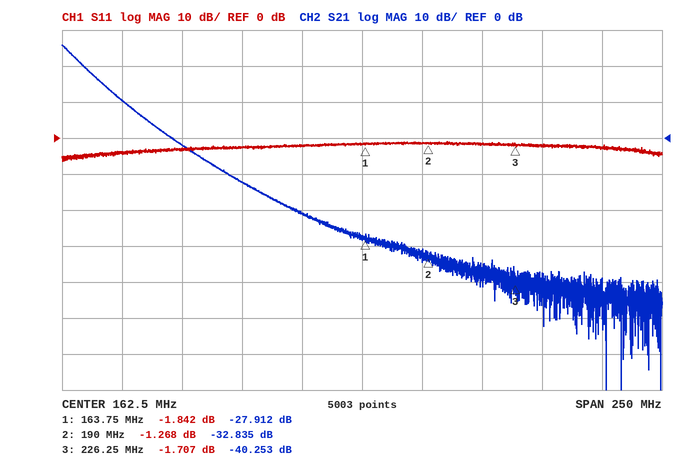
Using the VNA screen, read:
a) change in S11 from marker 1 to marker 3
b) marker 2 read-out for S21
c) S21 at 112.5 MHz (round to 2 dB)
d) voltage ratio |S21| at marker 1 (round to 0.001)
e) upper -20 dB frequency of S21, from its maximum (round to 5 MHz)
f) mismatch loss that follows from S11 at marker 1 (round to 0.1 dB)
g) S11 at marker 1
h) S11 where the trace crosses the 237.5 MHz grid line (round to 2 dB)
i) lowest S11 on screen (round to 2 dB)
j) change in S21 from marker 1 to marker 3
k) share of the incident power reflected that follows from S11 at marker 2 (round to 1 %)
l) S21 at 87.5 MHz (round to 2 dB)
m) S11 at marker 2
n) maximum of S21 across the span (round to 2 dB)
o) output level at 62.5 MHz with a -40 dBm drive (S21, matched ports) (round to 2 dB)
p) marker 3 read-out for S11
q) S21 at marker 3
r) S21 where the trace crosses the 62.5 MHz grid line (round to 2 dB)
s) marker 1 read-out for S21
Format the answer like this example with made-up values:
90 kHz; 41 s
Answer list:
0.135 dB; -32.835 dB; -12 dB; 0.040; 70 MHz; 4.6 dB; -1.842 dB; -2 dB; -6 dB; -12.341 dB; 75 %; -2 dB; -1.268 dB; 26 dB; -30 dBm; -1.707 dB; -40.253 dB; 10 dB; -27.912 dB
